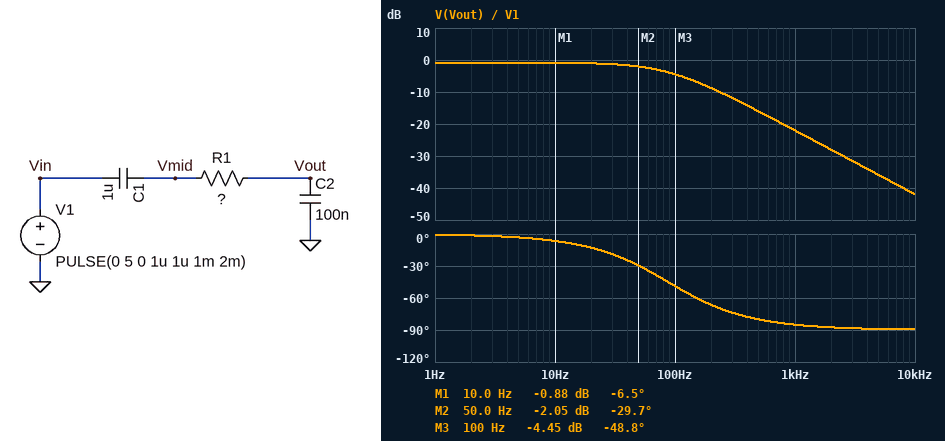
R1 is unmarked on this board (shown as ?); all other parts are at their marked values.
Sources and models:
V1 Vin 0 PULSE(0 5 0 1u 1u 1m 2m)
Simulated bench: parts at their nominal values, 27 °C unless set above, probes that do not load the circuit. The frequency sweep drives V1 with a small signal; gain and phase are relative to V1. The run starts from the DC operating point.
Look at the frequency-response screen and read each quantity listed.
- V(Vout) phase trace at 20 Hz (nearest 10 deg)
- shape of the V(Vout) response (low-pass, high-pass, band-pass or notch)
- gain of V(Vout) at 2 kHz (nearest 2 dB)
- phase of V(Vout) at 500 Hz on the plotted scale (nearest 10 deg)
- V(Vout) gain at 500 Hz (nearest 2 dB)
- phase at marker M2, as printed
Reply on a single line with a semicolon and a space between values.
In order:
-10 deg; low-pass; -28 dB; -80 deg; -16 dB; -29.7 deg
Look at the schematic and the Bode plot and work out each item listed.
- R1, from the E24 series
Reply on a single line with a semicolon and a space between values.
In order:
20 kΩ
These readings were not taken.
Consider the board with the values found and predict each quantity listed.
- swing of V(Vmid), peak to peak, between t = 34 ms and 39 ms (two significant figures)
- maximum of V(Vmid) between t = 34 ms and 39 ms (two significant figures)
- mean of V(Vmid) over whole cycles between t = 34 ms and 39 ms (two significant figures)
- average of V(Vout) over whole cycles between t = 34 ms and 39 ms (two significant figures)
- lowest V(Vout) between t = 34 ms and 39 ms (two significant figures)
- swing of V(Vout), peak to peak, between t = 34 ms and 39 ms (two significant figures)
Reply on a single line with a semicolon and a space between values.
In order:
5.1 V; 4.8 V; 2.3 V; 2.3 V; 1.7 V; 1.2 V
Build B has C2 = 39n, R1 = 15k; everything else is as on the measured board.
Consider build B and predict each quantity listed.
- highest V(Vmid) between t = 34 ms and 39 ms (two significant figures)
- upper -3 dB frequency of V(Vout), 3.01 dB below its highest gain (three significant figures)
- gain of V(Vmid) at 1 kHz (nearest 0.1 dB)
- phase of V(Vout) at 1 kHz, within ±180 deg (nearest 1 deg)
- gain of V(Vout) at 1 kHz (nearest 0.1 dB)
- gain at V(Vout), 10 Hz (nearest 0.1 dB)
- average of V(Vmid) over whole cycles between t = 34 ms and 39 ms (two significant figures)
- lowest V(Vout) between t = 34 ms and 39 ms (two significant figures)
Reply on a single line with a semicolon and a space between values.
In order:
5.0 V; 283 Hz; 0 dB; -74 deg; -11.6 dB; -0.3 dB; 2.4 V; 700 mV
